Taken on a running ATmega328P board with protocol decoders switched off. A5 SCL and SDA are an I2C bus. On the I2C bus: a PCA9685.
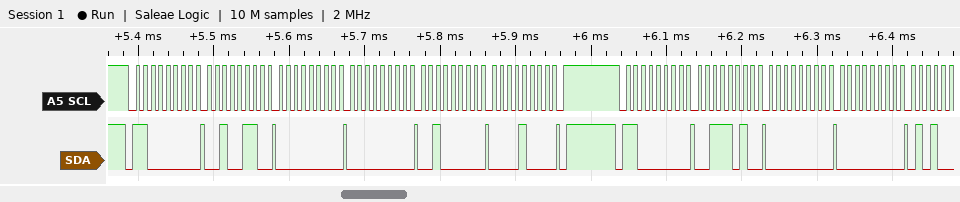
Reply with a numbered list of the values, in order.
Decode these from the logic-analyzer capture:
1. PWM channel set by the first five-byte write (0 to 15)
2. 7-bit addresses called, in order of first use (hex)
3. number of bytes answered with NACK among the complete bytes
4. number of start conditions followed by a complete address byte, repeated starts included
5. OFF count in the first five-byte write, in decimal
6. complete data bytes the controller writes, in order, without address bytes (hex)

1. 8
2. 0x60
3. 0
4. 2
5. 2080
6. 26 00 00 20 08 3A 00 00
